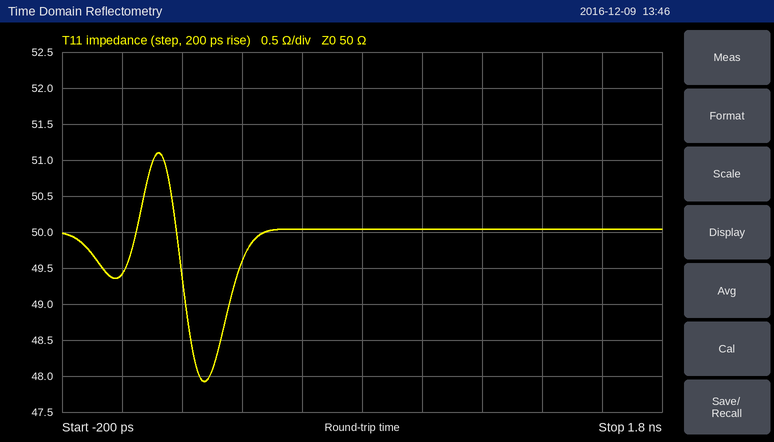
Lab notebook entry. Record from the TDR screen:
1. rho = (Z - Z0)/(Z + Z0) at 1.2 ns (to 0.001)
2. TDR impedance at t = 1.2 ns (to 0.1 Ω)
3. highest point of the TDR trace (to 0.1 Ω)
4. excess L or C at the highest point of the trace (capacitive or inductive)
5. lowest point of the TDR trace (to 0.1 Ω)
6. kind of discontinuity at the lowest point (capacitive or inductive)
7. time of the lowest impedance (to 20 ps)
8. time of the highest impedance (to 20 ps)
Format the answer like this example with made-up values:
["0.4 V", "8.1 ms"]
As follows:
["0.000", "50.0 Ω", "51.1 Ω", "inductive", "47.9 Ω", "capacitive", "280 ps", "120 ps"]
